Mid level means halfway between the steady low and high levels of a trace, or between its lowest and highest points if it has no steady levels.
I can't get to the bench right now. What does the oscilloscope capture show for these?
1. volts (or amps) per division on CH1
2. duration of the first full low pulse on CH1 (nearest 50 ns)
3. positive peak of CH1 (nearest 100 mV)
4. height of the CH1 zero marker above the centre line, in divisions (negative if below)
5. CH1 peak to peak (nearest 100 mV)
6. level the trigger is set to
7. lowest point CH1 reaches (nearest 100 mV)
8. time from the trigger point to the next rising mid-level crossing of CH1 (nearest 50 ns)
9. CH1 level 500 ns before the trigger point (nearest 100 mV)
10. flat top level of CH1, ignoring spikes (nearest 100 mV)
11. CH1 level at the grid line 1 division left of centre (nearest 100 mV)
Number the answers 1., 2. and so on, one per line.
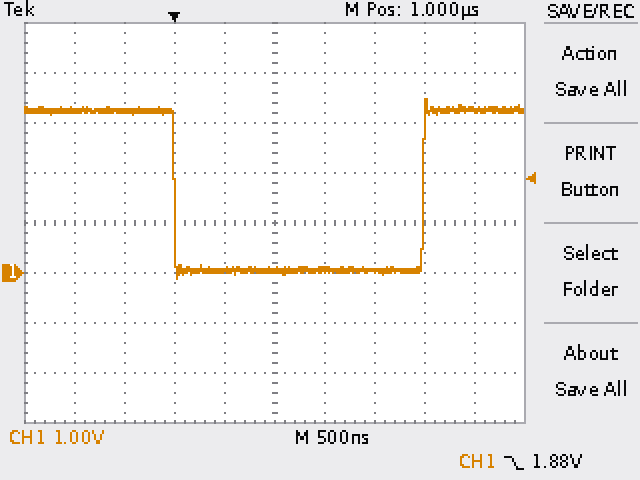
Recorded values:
1. 1 V
2. 2.50 µs
3. 3.5 V
4. -1.0 div
5. 3.6 V
6. 1.88 V
7. -100 mV
8. 2.50 µs
9. 3.2 V
10. 3.2 V
11. 100 mV
